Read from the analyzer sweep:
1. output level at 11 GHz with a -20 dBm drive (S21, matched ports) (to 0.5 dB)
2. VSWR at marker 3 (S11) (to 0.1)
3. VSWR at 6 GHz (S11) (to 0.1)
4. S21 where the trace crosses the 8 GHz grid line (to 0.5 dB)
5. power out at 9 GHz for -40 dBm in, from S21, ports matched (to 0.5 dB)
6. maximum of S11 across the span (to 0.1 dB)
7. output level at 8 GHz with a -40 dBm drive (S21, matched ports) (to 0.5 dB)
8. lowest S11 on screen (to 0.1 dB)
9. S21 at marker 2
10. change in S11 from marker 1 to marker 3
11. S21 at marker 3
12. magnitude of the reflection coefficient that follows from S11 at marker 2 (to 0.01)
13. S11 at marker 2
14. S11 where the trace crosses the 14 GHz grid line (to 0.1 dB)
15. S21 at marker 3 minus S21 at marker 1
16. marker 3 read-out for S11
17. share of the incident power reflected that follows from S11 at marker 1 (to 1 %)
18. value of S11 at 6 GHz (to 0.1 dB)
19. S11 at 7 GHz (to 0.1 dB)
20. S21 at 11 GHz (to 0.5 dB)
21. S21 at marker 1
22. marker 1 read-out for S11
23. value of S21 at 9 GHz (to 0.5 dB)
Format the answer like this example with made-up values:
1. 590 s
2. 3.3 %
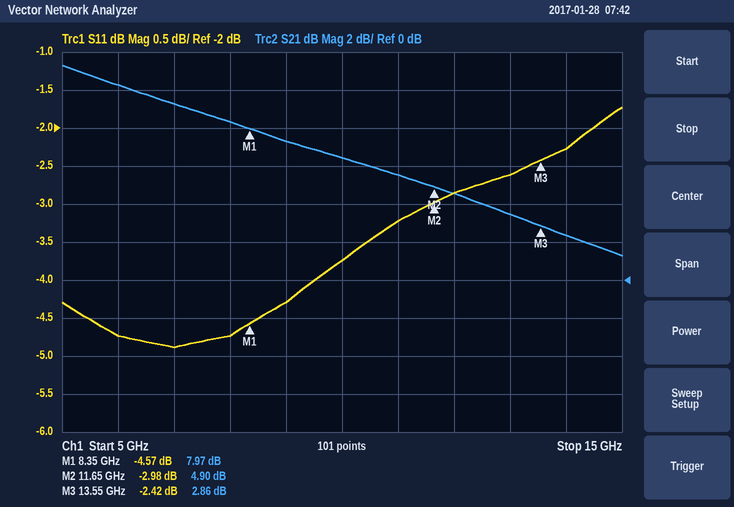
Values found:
1. -14.5 dBm
2. 7.2
3. 3.8
4. 8.5 dB
5. -32.5 dBm
6. -1.7 dB
7. -31.5 dBm
8. -4.9 dB
9. 4.90 dB
10. 2.15 dB
11. 2.86 dB
12. 0.71
13. -2.98 dB
14. -2.3 dB
15. -5.11 dB
16. -2.42 dB
17. 35 %
18. -4.7 dB
19. -4.9 dB
20. 5.5 dB
21. 7.97 dB
22. -4.57 dB
23. 7.5 dB
